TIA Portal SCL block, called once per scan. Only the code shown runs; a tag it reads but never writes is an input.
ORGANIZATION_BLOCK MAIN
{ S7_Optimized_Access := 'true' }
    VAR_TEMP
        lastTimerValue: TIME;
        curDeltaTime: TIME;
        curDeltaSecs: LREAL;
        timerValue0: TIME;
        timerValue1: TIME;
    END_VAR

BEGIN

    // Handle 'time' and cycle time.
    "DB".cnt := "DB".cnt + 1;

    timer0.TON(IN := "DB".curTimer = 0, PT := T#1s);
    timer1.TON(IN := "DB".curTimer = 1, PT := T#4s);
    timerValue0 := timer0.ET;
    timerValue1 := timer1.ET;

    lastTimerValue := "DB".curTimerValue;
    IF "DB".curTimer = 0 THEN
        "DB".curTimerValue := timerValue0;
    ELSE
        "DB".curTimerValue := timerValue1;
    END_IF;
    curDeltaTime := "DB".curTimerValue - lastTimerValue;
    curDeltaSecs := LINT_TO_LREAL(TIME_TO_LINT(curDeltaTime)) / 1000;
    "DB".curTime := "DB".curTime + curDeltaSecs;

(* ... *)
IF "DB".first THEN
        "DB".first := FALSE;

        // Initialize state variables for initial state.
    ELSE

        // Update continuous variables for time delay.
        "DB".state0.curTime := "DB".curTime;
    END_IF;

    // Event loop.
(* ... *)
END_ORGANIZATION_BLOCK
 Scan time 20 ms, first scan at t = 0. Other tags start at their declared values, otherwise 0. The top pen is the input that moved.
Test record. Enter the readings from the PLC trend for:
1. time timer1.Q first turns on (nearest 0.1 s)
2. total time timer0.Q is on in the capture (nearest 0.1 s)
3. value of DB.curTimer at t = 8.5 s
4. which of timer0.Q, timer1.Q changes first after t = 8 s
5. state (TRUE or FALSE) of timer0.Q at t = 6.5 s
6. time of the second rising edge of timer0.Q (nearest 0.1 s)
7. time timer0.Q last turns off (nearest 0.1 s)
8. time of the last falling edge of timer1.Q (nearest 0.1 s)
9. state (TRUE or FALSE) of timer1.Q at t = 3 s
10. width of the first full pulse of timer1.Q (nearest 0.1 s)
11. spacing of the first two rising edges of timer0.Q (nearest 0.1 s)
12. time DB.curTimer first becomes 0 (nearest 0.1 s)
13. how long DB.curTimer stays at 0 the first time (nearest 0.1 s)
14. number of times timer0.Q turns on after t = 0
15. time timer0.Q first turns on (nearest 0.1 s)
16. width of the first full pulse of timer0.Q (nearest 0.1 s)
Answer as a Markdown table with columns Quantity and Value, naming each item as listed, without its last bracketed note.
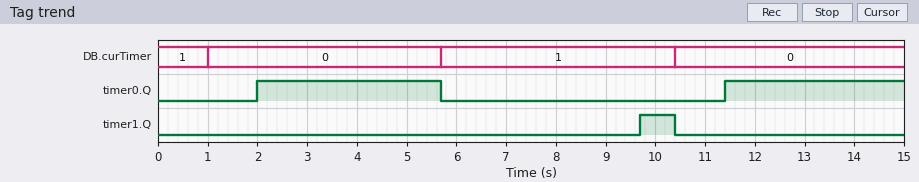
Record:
| Quantity | Value |
|---|---|
| time timer1.Q first turns on | 9.7 s |
| total time timer0.Q is on in the capture | 7.3 s |
| value of DB.curTimer at t = 8.5 s | 1 |
| which of timer0.Q, timer1.Q changes first after t = 8 s | timer1.Q |
| state (TRUE or FALSE) of timer0.Q at t = 6.5 s | FALSE |
| time of the second rising edge of timer0.Q | 11.4 s |
| time timer0.Q last turns off | 5.7 s |
| time of the last falling edge of timer1.Q | 10.4 s |
| state (TRUE or FALSE) of timer1.Q at t = 3 s | FALSE |
| width of the first full pulse of timer1.Q | 0.7 s |
| spacing of the first two rising edges of timer0.Q | 9.4 s |
| time DB.curTimer first becomes 0 | 1.0 s |
| how long DB.curTimer stays at 0 the first time | 4.7 s |
| number of times timer0.Q turns on after t = 0 | 2 |
| time timer0.Q first turns on | 2.0 s |
| width of the first full pulse of timer0.Q | 3.7 s |
